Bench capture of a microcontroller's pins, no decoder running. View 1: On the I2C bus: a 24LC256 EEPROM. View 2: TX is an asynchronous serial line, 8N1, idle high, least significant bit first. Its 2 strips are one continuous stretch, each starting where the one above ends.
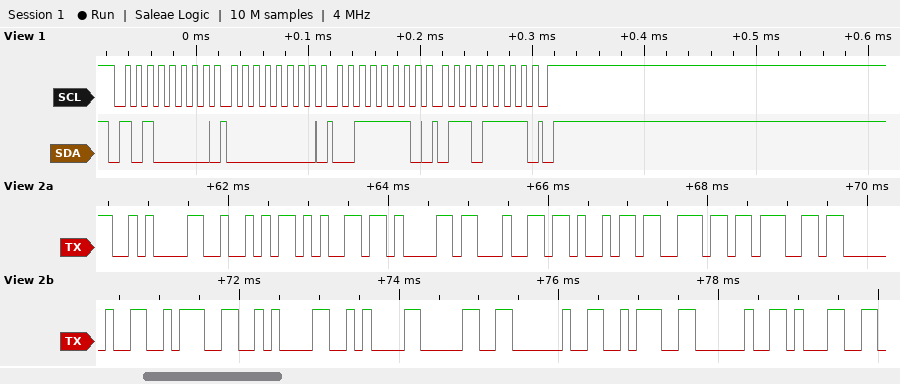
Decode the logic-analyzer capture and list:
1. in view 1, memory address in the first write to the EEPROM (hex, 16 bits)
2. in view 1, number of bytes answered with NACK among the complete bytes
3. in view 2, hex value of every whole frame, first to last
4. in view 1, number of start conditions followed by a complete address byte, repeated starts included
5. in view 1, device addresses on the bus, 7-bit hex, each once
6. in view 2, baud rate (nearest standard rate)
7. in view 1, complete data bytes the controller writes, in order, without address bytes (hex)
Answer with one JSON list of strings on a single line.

["0x003E", "0", "0A 52 65 61 64 69 6E 67 20 3A 0A 0A 30 20 3A 20 31", "1", "0x50", "9600 baud", "00 3E 6F"]
